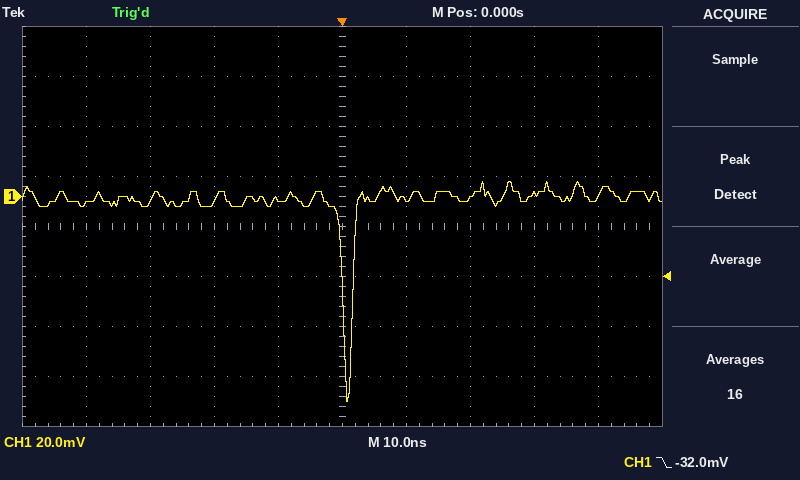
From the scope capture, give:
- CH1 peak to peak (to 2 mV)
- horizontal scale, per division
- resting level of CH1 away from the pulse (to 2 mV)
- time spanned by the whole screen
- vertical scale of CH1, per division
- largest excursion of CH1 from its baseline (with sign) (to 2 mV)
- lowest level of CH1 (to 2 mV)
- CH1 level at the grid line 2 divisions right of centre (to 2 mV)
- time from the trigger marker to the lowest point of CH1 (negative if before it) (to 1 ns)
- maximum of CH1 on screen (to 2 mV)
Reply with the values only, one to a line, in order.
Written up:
88 mV
10 ns
-2 mV
100 ns
20 mV
-80 mV
-82 mV
0 mV
+1 ns
6 mV
